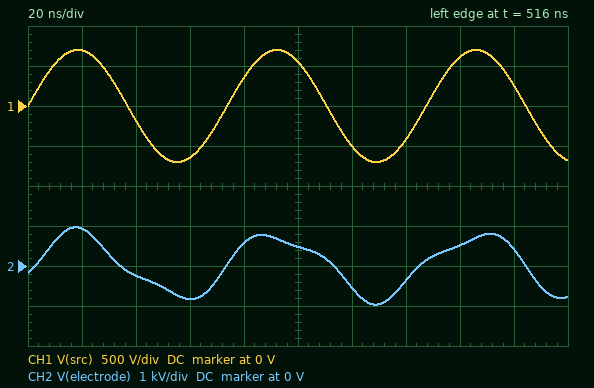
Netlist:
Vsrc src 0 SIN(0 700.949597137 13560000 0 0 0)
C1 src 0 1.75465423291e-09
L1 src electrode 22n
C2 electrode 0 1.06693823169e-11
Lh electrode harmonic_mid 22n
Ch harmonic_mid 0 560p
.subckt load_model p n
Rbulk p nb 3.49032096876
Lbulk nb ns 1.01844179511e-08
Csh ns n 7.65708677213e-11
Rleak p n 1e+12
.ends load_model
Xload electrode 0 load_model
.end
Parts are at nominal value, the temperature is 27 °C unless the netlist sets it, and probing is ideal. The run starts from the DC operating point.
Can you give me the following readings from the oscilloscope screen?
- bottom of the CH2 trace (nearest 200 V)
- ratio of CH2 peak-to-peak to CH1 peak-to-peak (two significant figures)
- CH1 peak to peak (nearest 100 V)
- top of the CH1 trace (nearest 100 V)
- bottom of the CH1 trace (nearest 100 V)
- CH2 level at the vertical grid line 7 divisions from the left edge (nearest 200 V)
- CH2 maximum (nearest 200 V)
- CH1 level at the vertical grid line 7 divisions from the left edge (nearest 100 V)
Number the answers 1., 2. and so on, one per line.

1. -1.0 kV
2. 1.4
3. 1.4 kV
4. 700 V
5. -700 V
6. -400 V
7. 1.0 kV
8. -400 V
